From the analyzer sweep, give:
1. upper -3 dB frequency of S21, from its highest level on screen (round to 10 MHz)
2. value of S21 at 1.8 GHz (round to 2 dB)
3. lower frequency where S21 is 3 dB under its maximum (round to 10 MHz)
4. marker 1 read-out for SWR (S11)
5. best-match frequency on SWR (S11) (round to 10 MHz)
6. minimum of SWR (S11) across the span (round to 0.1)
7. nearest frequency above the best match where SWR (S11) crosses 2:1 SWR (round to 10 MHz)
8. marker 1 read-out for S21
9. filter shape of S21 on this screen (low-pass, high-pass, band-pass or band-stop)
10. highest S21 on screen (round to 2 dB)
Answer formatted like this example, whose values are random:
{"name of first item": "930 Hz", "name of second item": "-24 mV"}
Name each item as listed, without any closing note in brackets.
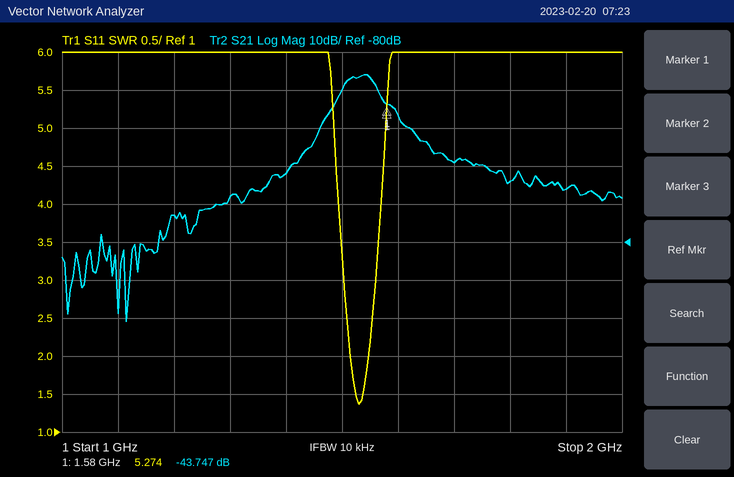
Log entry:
{"upper -3 dB frequency of S21, from its highest level on screen": "1.56 GHz", "value of S21 at 1.8 GHz": "-64 dB", "lower frequency where S21 is 3 dB under its maximum": "1.50 GHz", "marker 1 read-out for SWR": "5.274", "best-match frequency on SWR (S11)": "1.53 GHz", "minimum of SWR (S11) across the span": "1.4", "nearest frequency above the best match where SWR (S11) crosses 2:1 SWR": "1.55 GHz", "marker 1 read-out for S21": "-43.747 dB", "filter shape of S21 on this screen": "band-pass", "highest S21 on screen": "-36 dB"}
